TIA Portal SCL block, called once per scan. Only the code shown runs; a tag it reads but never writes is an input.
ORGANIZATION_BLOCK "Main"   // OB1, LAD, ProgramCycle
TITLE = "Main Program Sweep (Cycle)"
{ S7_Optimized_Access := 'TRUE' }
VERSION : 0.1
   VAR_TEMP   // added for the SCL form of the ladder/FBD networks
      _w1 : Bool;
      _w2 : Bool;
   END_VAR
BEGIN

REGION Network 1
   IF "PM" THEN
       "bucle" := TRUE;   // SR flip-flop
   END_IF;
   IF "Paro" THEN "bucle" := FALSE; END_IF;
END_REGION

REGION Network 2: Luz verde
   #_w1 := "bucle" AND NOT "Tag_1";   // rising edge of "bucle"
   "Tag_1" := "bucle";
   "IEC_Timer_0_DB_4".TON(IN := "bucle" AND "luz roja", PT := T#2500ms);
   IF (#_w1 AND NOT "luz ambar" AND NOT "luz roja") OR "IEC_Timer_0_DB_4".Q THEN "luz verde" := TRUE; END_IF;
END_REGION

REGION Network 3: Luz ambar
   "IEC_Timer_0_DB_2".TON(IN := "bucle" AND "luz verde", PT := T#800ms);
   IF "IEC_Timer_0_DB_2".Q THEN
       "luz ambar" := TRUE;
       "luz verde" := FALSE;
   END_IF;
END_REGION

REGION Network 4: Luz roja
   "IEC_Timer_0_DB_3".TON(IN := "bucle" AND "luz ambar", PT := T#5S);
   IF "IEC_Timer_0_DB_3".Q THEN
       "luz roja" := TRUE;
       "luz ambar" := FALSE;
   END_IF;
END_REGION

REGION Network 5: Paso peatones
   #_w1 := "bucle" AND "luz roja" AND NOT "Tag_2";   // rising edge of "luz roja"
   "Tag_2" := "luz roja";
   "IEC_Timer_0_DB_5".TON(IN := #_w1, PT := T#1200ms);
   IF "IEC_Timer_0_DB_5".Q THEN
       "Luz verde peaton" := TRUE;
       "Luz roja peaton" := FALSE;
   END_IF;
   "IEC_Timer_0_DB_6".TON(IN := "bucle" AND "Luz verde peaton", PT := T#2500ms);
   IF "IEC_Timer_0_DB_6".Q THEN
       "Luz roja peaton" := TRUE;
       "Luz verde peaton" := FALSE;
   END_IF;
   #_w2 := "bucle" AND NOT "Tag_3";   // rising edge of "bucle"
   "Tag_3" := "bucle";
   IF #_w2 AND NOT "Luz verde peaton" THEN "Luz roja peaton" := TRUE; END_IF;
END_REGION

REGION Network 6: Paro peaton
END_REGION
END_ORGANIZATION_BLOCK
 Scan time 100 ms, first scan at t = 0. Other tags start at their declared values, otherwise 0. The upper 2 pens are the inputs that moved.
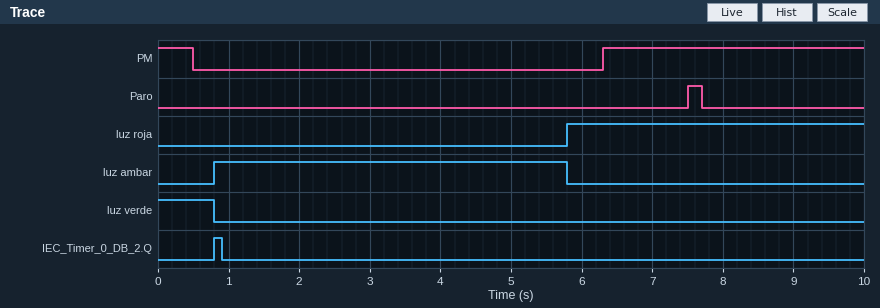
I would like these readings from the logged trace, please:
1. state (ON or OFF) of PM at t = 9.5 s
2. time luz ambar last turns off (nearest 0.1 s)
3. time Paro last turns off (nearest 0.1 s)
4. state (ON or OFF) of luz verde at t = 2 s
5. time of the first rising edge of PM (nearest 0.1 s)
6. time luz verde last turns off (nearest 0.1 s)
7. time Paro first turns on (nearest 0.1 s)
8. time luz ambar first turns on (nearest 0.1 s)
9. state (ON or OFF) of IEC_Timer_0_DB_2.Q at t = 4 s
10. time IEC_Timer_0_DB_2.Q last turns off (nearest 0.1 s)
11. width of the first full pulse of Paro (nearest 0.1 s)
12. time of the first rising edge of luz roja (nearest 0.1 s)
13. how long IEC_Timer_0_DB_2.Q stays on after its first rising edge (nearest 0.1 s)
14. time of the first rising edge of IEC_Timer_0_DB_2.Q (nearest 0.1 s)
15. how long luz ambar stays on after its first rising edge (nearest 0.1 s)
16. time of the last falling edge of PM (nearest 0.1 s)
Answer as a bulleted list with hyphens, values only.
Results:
- ON
- 5.8 s
- 7.7 s
- OFF
- 6.3 s
- 0.8 s
- 7.5 s
- 0.8 s
- OFF
- 0.9 s
- 0.2 s
- 5.8 s
- 0.1 s
- 0.8 s
- 5.0 s
- 0.5 s
